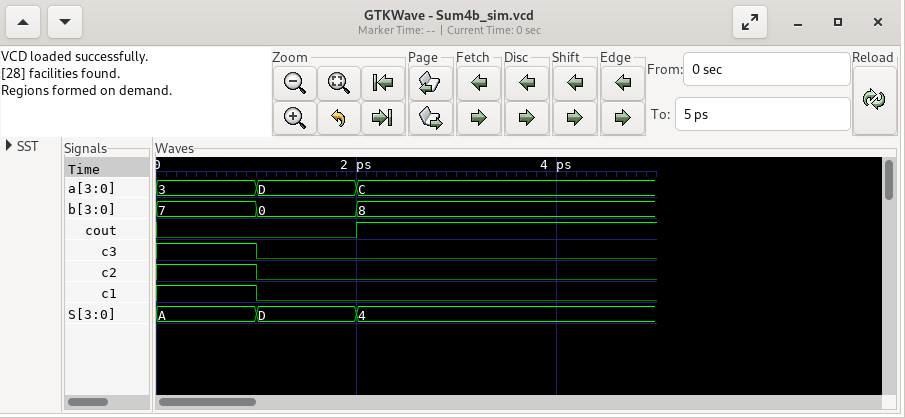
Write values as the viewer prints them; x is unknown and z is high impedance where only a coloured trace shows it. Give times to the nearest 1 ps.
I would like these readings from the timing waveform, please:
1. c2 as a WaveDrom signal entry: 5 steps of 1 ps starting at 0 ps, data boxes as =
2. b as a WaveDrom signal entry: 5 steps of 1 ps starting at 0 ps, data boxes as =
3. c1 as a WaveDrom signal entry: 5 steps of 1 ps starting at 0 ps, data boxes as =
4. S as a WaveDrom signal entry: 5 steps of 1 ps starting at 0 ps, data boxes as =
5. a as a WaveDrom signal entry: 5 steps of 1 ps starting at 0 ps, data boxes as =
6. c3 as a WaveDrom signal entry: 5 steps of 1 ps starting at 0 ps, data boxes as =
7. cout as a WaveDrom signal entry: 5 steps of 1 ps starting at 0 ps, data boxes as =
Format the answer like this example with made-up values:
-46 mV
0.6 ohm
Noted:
{name: 'c2', wave: '10...'}
{name: 'b', wave: '===..', data: '7 0 8'}
{name: 'c1', wave: '10...'}
{name: 'S', wave: '===..', data: 'A D 4'}
{name: 'a', wave: '===..', data: '3 D C'}
{name: 'c3', wave: '10...'}
{name: 'cout', wave: '0.1..'}
